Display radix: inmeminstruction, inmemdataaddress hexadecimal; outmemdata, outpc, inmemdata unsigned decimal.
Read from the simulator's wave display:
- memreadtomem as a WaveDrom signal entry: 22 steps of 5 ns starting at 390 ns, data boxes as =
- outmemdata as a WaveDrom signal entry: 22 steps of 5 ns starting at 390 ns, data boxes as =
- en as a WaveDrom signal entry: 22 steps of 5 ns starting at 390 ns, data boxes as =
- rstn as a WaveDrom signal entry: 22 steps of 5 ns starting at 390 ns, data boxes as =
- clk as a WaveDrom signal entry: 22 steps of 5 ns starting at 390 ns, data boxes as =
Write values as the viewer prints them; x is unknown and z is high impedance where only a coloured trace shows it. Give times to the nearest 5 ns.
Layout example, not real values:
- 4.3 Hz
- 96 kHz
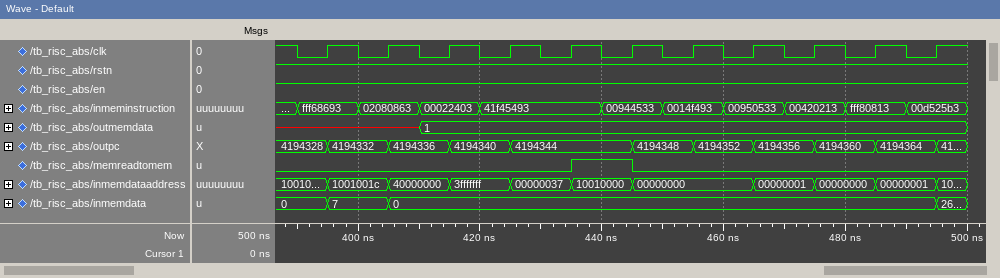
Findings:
- {name: 'memreadtomem', wave: '0........1.0..........'}
- {name: 'outmemdata', wave: 'x...=.................', data: '1'}
- {name: 'en', wave: '1.....................'}
- {name: 'rstn', wave: '1.....................'}
- {name: 'clk', wave: '0101010101010101010101'}
